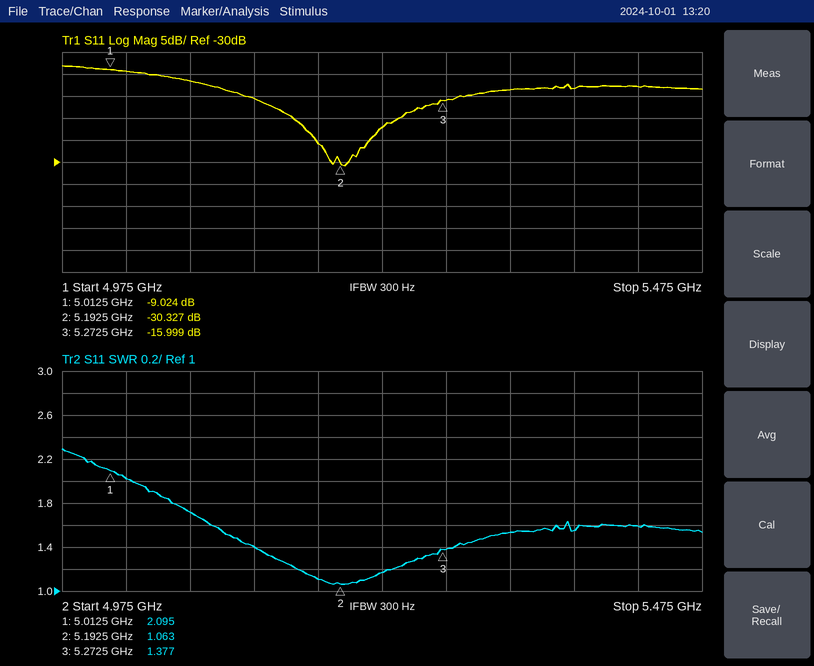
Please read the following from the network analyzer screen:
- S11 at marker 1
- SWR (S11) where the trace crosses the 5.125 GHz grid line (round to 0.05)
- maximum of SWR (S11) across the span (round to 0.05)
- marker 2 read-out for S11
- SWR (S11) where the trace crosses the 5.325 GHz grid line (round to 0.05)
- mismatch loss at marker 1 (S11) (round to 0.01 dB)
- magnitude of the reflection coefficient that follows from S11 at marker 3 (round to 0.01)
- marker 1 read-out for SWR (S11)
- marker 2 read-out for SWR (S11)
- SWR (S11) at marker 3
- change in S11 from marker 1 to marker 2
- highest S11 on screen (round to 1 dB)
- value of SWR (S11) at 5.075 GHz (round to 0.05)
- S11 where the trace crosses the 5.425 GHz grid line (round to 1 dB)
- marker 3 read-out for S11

-9.024 dB
1.40
2.30
-30.327 dB
1.55
0.58 dB
0.16
2.095
1.063
1.377
-21.303 dB
-8 dB
1.70
-13 dB
-15.999 dB
